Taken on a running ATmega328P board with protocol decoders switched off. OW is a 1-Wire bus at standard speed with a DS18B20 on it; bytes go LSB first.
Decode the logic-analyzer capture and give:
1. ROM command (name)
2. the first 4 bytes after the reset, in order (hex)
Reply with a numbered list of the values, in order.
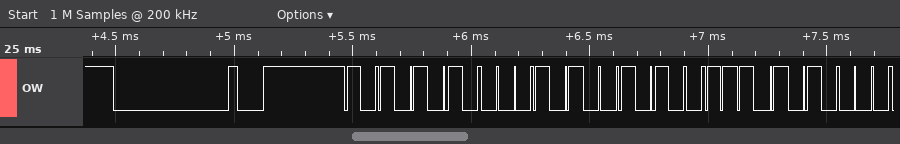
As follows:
1. Match ROM
2. 55 28 E5 0A
